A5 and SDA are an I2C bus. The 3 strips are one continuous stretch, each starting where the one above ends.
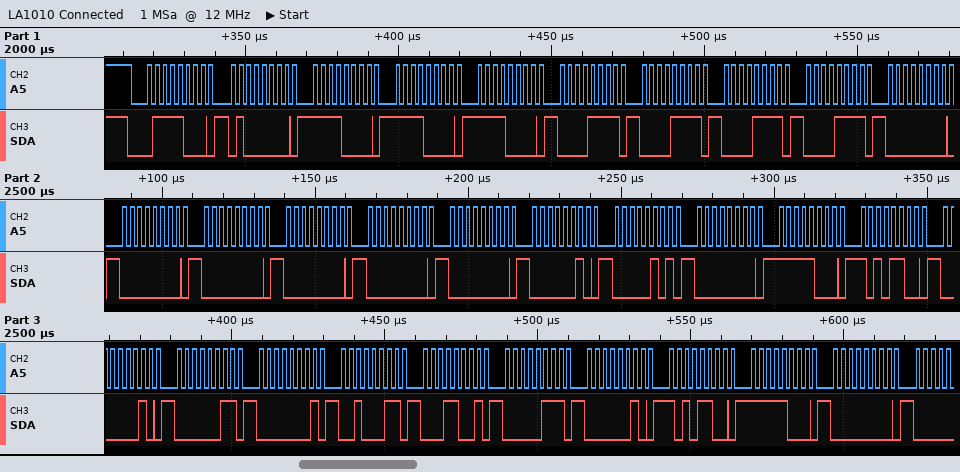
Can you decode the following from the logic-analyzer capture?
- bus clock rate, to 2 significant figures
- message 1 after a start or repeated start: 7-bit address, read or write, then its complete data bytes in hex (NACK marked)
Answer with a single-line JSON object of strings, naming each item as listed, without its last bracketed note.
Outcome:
{"bus clock rate, to 2 significant figures": "400 kHz", "message 1 after a start or repeated start: 7-bit address, read or write, then its complete data bytes in hex": "0x3C write: 40 F0 F0 F0 0F 0F 0F 0F 00 00 00 00 00 00 02 05 00 F8 AC 02 03 01 23 19 07 02 AC F8 00"}
